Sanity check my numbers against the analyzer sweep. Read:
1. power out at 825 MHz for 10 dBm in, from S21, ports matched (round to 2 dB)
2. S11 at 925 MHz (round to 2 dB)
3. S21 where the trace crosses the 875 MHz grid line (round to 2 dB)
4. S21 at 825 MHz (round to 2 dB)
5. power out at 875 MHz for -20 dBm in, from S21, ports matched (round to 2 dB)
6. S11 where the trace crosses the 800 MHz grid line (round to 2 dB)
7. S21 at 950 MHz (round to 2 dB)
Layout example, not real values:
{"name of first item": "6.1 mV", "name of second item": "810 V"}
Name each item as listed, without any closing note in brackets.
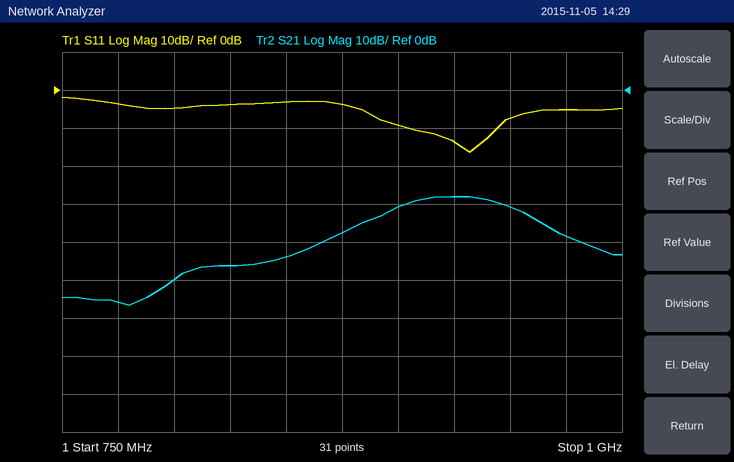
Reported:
{"power out at 825 MHz for 10 dBm in, from S21, ports matched": "-36 dBm", "S11 at 925 MHz": "-14 dB", "S21 where the trace crosses the 875 MHz grid line": "-38 dB", "S21 at 825 MHz": "-46 dB", "power out at 875 MHz for -20 dBm in, from S21, ports matched": "-58 dBm", "S11 where the trace crosses the 800 MHz grid line": "-4 dB", "S21 at 950 MHz": "-30 dB"}
